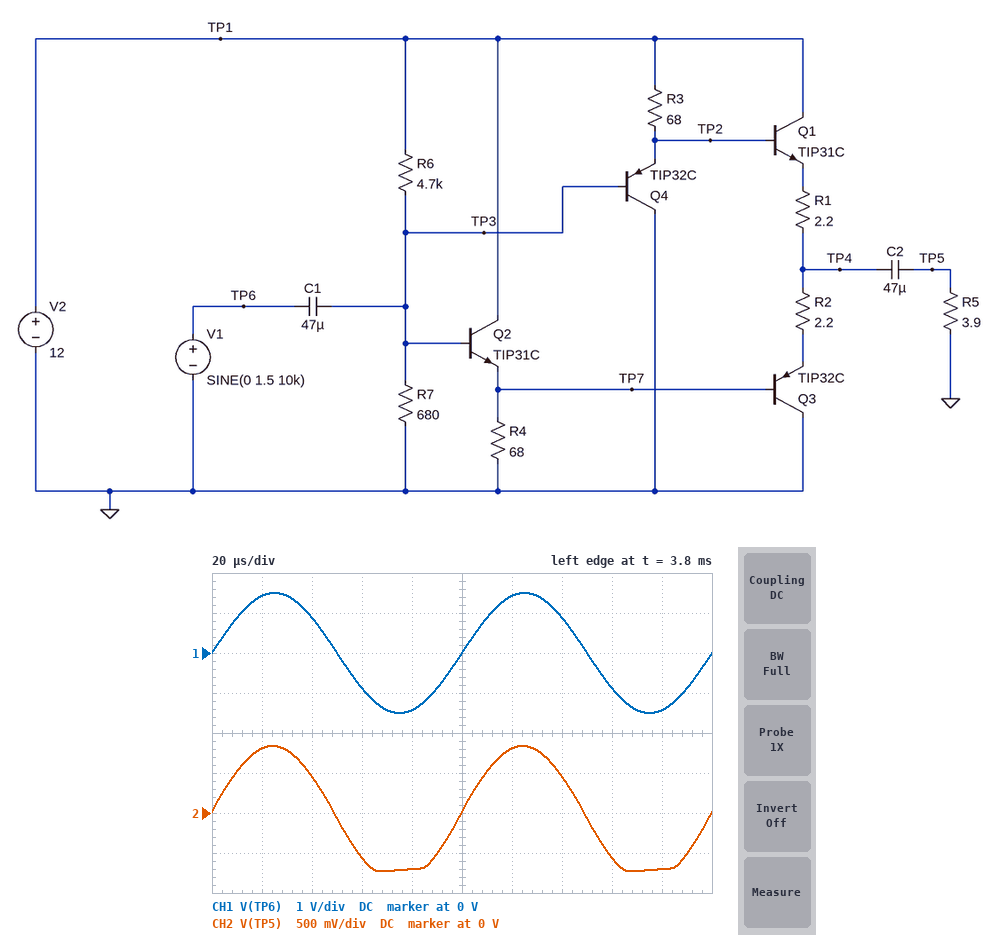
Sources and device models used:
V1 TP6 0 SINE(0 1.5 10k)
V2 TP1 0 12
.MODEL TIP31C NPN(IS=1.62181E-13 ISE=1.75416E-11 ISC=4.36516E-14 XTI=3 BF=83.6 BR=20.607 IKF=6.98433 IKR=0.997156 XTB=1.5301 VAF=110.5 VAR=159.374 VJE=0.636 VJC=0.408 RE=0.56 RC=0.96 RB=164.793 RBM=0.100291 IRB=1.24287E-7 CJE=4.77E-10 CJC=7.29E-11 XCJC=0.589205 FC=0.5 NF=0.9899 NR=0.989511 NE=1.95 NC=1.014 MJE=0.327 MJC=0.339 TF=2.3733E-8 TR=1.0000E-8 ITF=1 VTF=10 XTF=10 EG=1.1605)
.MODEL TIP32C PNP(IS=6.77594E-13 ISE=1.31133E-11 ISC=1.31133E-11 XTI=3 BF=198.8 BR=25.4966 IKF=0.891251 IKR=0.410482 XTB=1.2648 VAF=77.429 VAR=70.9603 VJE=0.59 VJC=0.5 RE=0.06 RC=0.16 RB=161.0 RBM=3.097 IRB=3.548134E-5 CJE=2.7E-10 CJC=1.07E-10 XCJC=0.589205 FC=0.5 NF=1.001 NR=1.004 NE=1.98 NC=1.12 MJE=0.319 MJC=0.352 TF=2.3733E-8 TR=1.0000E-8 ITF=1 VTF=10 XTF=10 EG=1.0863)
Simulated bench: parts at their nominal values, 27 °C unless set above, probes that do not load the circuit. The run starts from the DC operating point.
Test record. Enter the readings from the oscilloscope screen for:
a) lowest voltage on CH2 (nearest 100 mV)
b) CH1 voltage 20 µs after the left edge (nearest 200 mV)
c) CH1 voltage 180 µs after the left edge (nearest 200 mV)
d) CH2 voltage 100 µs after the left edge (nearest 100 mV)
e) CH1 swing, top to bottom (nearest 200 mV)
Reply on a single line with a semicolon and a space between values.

-700 mV; 1.4 V; -1.4 V; 0 V; 3.0 V
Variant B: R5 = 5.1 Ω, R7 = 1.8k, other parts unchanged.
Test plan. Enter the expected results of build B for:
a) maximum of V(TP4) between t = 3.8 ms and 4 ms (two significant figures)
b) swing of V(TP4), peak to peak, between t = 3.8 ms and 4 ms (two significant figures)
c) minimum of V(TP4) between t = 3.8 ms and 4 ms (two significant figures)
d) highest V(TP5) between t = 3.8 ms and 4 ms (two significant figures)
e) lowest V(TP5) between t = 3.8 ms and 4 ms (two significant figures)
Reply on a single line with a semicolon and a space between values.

4.5 V; 2.0 V; 2.5 V; 970 mV; -980 mV
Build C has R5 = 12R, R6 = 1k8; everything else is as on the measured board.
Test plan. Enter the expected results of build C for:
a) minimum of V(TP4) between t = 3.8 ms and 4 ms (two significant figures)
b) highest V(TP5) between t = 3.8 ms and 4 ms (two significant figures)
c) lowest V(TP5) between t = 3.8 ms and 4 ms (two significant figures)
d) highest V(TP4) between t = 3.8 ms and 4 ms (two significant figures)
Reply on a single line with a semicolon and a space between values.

2.1 V; 1.2 V; -1.2 V; 4.6 V
